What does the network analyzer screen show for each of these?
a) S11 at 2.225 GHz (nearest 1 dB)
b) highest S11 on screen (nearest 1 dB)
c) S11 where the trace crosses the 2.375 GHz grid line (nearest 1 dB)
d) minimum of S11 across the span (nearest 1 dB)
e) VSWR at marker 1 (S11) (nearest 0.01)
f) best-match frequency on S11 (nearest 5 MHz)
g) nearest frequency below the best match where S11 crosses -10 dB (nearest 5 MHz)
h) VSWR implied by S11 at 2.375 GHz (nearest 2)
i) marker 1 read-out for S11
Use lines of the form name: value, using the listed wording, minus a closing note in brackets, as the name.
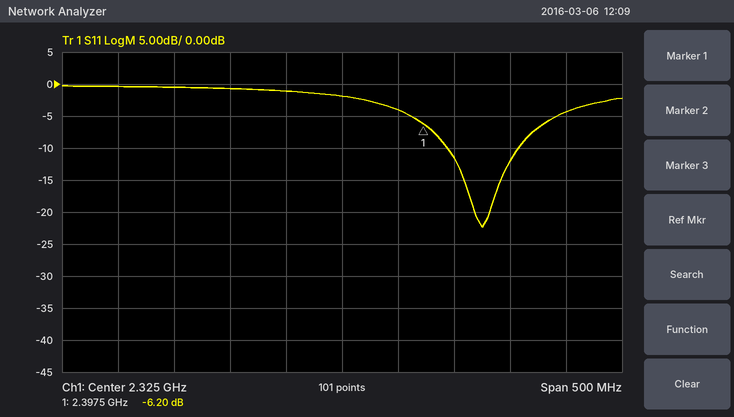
S11 at 2.225 GHz: -1 dB
highest S11 on screen: 0 dB
S11 where the trace crosses the 2.375 GHz grid line: -4 dB
minimum of S11 across the span: -22 dB
VSWR at marker 1 (S11): 2.92
best-match frequency on S11: 2.450 GHz
nearest frequency below the best match where S11 crosses -10 dB: 2.420 GHz
VSWR implied by S11 at 2.375 GHz: 4
marker 1 read-out for S11: -6.20 dB
